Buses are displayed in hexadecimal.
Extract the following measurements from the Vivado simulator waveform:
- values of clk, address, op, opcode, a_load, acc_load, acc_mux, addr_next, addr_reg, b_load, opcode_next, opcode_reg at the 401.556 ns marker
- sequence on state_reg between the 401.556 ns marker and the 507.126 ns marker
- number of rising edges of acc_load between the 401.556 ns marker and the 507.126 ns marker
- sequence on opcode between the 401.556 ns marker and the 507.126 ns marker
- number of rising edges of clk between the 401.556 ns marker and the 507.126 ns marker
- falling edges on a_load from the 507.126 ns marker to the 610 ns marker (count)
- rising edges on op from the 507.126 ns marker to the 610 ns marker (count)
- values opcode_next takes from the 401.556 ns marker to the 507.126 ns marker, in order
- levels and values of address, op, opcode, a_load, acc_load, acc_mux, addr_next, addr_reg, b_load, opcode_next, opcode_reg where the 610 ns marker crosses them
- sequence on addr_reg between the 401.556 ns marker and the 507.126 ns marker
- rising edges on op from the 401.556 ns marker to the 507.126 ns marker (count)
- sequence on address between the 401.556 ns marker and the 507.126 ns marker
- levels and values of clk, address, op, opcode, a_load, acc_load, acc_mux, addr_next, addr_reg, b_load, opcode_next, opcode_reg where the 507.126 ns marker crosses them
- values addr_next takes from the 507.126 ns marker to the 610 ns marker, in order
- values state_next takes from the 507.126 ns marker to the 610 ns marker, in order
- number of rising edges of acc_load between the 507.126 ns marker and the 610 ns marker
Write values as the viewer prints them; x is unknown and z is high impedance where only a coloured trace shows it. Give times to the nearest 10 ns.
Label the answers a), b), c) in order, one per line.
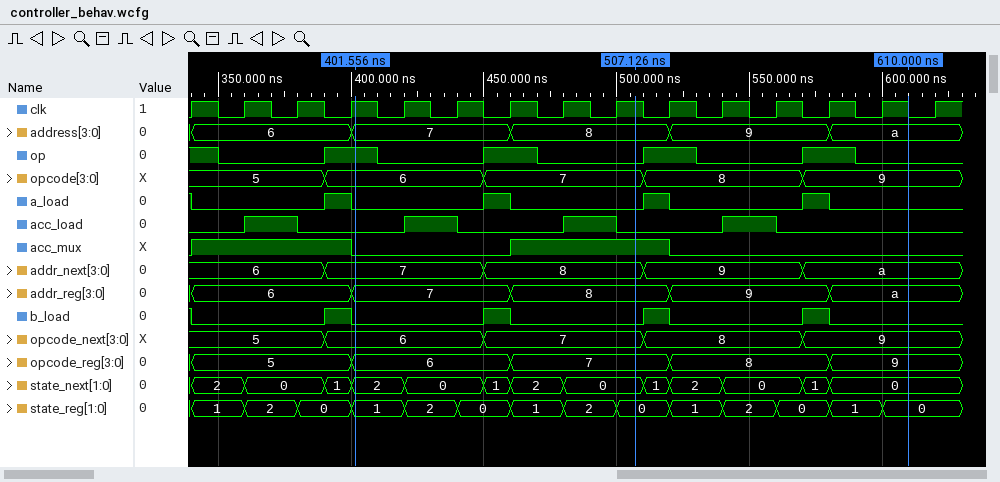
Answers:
a) clk=1, address=7, op=1, opcode=6, a_load=0, acc_load=0, acc_mux=0, addr_next=7, addr_reg=7, b_load=0, opcode_next=6, opcode_reg=6
b) 1, 2, 0, 1, 2, 0
c) 2
d) 6, 7
e) 5
f) 2
g) 2
h) 6, 7
i) address=a, op=0, opcode=9, a_load=0, acc_load=0, acc_mux=0, addr_next=a, addr_reg=a, b_load=0, opcode_next=9, opcode_reg=9
j) 7, 8
k) 1
l) 7, 8
m) clk=1, address=8, op=0, opcode=7, a_load=0, acc_load=0, acc_mux=1, addr_next=8, addr_reg=8, b_load=0, opcode_next=7, opcode_reg=7
n) 8, 9, a
o) 0, 1, 2, 0, 1, 0
p) 1
